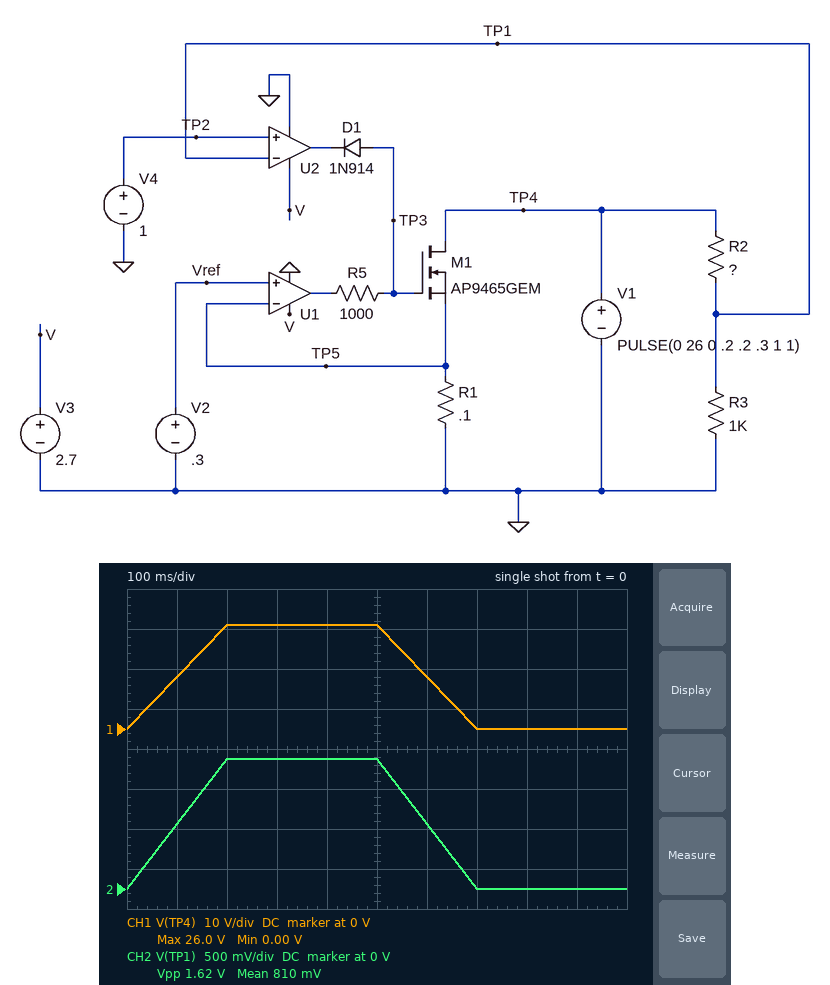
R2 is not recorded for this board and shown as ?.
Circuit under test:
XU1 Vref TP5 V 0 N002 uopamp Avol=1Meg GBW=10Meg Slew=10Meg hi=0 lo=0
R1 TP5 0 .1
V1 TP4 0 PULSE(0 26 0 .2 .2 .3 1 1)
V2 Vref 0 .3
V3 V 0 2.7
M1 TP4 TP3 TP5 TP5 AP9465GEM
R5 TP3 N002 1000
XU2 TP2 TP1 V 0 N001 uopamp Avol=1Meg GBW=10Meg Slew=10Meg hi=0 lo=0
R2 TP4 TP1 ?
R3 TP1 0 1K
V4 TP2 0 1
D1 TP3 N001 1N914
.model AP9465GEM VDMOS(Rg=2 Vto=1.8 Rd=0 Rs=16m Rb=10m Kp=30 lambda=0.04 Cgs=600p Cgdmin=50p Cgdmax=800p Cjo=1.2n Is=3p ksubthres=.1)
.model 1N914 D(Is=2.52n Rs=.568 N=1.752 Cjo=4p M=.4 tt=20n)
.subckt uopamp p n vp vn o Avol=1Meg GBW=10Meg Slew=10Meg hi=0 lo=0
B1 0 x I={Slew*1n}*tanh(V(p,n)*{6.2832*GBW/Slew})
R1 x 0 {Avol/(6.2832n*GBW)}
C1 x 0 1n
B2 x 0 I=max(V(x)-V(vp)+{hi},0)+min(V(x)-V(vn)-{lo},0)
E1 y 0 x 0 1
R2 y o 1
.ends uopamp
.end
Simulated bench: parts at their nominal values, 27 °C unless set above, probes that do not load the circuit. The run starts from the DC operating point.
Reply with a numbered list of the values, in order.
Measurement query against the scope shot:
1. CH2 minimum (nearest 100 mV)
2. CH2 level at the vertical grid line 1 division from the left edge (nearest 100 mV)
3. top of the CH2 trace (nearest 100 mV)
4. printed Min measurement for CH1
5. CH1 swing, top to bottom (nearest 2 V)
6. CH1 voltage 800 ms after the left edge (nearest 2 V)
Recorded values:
1. 0 V
2. 800 mV
3. 1.6 V
4. 0.00 V
5. 26 V
6. 0 V
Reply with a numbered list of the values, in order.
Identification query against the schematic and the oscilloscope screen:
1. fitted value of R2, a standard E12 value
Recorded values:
1. 15 kΩ
